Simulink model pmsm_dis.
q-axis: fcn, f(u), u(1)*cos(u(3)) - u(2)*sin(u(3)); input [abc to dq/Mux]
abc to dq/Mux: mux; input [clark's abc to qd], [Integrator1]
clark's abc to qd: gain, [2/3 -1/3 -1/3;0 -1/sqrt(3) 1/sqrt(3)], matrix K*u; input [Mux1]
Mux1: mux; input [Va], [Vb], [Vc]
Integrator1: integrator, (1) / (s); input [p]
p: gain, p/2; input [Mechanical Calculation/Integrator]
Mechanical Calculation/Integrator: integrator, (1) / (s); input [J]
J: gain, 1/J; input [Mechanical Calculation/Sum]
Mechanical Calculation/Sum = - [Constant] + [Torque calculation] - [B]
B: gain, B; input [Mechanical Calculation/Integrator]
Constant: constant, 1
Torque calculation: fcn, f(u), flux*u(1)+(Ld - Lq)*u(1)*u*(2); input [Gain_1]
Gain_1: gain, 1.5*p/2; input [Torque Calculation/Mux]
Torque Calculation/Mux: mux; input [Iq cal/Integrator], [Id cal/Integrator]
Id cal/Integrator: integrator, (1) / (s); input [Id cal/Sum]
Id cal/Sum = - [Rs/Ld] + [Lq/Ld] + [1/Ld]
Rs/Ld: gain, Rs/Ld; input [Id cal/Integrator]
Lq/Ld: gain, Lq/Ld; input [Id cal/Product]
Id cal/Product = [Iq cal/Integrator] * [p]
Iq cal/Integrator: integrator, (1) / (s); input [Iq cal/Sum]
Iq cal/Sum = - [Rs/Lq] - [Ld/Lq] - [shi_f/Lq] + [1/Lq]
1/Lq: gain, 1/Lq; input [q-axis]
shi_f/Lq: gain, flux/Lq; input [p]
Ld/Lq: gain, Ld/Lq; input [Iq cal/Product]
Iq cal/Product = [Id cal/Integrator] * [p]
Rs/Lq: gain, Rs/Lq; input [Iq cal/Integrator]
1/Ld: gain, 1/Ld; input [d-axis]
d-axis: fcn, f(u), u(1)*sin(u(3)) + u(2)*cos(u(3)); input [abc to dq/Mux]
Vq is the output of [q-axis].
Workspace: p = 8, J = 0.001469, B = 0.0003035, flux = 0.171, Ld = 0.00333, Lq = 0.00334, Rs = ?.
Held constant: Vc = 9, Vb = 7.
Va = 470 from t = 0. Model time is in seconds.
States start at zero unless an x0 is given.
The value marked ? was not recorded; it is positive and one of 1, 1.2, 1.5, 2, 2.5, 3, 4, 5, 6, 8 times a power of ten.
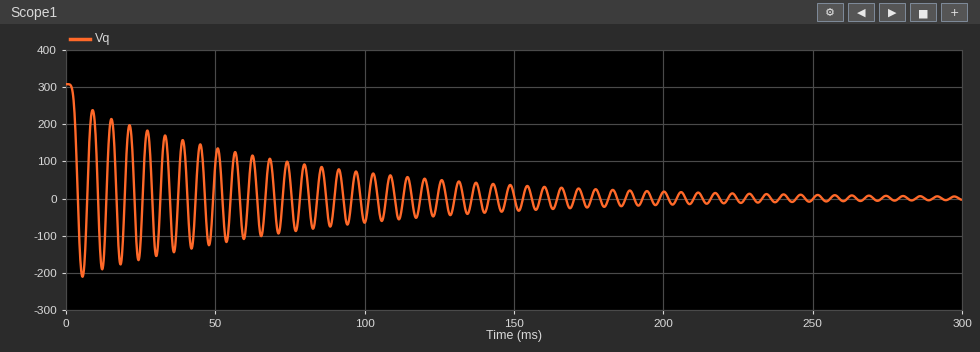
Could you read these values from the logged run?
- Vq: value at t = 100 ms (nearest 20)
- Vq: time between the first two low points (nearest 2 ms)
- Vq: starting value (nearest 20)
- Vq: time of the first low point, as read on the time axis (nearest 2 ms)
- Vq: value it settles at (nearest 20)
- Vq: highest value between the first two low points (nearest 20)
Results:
-60
6 ms
300
6 ms
0
240
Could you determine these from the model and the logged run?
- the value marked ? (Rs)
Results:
0.8
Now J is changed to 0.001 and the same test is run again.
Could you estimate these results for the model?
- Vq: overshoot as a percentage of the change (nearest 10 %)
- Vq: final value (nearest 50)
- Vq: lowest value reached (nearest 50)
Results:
70 %
0
-200
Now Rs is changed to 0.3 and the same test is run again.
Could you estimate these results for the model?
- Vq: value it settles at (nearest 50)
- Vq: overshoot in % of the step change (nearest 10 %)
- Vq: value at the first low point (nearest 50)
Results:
0
70 %
-200
